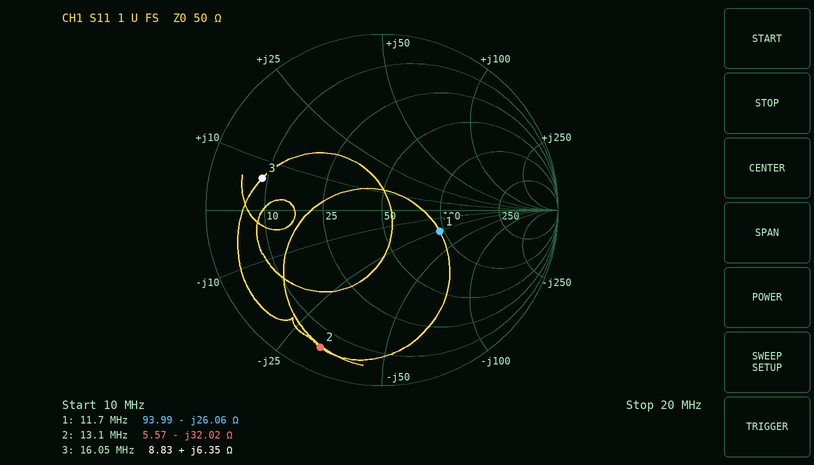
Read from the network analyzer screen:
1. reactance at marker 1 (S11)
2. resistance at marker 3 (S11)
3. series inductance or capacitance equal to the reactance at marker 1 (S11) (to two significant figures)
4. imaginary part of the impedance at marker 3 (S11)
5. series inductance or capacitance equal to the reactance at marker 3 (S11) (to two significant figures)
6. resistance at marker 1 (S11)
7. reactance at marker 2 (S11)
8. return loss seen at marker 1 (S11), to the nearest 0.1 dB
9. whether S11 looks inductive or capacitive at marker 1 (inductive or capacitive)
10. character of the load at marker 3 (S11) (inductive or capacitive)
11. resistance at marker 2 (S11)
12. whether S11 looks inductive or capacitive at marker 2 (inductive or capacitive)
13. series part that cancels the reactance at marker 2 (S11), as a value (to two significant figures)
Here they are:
-26.06 Ω
8.83 Ω
520 pF
+6.35 Ω
63 nH
93.99 Ω
-32.02 Ω
9.1 dB
capacitive
inductive
5.57 Ω
capacitive
390 nH
